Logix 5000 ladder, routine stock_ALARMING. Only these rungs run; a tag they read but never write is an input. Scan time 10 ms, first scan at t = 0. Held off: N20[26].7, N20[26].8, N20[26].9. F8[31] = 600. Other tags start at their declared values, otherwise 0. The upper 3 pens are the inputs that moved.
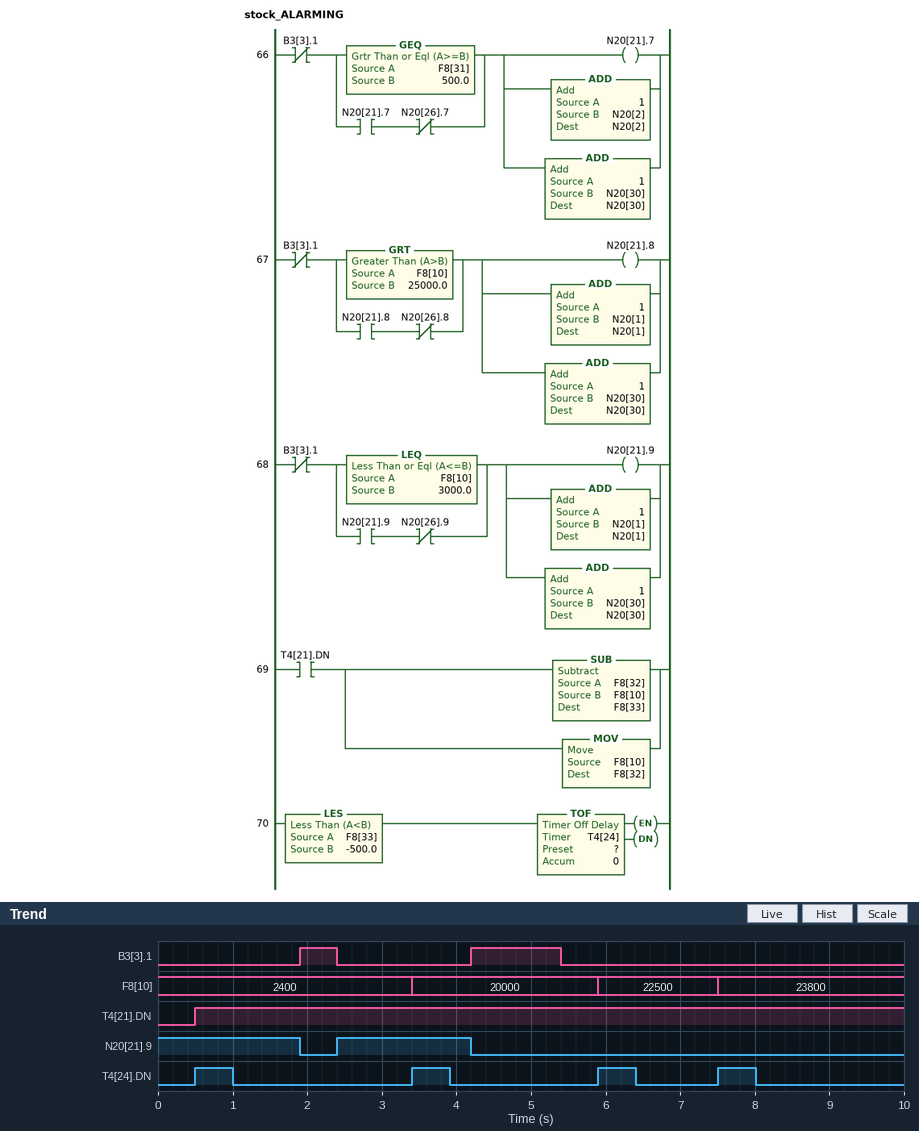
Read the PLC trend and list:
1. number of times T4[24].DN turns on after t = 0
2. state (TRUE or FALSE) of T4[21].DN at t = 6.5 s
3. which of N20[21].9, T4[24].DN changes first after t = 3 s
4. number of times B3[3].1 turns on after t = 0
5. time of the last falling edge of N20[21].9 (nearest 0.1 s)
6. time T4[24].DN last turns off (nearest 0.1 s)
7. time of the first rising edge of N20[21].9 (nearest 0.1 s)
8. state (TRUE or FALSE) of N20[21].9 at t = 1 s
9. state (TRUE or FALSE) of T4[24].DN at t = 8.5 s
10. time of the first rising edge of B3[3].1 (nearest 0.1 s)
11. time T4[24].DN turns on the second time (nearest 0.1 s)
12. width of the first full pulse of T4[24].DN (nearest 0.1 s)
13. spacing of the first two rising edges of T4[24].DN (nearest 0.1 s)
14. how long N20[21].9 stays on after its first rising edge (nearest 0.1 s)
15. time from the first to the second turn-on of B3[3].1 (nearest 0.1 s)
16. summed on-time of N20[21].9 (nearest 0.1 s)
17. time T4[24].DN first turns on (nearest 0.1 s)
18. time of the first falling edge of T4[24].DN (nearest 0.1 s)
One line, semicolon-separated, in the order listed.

4; TRUE; T4[24].DN; 2; 4.2 s; 8.0 s; 2.4 s; TRUE; FALSE; 1.9 s; 3.4 s; 0.5 s; 2.9 s; 1.8 s; 2.3 s; 3.7 s; 0.5 s; 1.0 s
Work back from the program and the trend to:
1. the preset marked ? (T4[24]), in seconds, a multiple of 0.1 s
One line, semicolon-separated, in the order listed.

0.5 s
